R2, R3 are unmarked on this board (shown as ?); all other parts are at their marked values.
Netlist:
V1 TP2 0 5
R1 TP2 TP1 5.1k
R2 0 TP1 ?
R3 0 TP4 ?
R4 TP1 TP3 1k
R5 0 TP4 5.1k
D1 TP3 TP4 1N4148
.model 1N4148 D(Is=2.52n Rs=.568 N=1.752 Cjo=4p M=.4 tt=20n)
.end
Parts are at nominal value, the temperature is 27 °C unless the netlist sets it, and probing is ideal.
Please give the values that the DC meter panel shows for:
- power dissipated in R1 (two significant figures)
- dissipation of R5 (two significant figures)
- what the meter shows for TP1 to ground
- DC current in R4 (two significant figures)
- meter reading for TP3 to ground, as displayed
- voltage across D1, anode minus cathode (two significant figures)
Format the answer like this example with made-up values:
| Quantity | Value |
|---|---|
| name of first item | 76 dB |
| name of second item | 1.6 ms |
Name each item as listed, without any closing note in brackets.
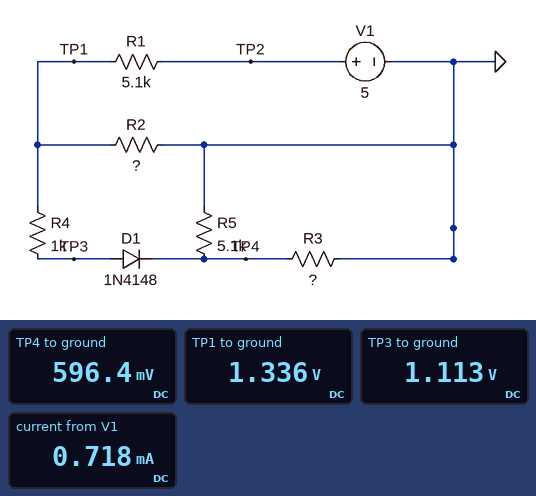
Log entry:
| Quantity | Value |
|---|---|
| power dissipated in R1 | 2.6 mW |
| dissipation of R5 | 70 µW |
| what the meter shows for TP1 to ground | 1.336 V |
| DC current in R4 | 220 µA |
| meter reading for TP3 to ground, as displayed | 1.113 V |
| voltage across D1, anode minus cathode | 520 mV |
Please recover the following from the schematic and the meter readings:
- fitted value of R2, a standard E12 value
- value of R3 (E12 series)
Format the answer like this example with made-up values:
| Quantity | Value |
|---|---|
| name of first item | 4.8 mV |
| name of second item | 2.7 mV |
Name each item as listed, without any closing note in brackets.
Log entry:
| Quantity | Value |
|---|---|
| fitted value of R2, a standard E12 value | 2.7 kΩ |
| value of R3 | 5.6 kΩ |
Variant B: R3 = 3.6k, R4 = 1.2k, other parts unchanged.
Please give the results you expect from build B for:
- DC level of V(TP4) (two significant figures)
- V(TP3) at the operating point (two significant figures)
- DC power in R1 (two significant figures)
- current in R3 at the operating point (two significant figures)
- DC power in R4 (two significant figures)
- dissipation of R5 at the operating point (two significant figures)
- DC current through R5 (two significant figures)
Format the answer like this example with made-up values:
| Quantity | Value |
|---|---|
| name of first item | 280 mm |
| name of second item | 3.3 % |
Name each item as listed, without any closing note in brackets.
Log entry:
| Quantity | Value |
|---|---|
| DC level of V(TP4) | 500 mV |
| V(TP3) at the operating point | 1.0 V |
| DC power in R1 | 2.7 mW |
| current in R3 at the operating point | 140 µA |
| DC power in R4 | 68 µW |
| dissipation of R5 at the operating point | 50 µW |
| DC current through R5 | 99 µA |
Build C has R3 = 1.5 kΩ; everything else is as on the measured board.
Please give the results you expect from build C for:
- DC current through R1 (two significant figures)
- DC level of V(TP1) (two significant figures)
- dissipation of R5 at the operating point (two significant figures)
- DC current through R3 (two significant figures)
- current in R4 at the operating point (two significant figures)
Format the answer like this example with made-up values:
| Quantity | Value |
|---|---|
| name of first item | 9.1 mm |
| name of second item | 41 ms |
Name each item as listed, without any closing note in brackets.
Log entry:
| Quantity | Value |
|---|---|
| DC current through R1 | 750 µA |
| DC level of V(TP1) | 1.2 V |
| dissipation of R5 at the operating point | 25 µW |
| DC current through R3 | 240 µA |
| current in R4 at the operating point | 310 µA |
